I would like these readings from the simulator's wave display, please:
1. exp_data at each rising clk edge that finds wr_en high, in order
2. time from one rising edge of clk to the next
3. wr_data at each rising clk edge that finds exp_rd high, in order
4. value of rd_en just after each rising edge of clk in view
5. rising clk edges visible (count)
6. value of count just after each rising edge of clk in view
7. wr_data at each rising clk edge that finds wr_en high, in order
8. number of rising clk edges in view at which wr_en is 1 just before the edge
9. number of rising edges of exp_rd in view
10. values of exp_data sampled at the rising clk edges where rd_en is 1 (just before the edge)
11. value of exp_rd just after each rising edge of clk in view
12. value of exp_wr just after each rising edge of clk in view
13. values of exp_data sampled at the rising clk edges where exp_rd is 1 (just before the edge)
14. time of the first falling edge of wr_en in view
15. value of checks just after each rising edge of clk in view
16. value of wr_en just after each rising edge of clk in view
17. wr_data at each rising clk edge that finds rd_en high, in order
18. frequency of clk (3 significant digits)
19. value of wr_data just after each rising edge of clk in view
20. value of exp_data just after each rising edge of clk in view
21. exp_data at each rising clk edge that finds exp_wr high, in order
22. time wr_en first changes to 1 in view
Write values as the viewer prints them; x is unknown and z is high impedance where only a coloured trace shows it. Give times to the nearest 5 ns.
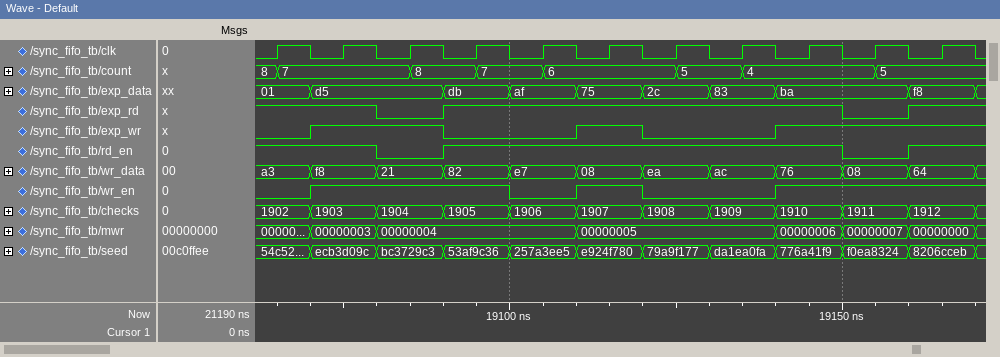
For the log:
d5, d5, db, 75, ba, ba, f8
10 ns
a3, f8, 82, e7, 08, ea, ac, 76, 64
1 1 0 1 1 1 1 1 1 0 1
11
7, 7, 8, 7, 6, 6, 5, 4, 4, 5, 5
f8, 21, 82, 08, 76, 08, 64
7
2
01, d5, db, af, 75, 2c, 83, ba, f8
1 1 0 1 1 1 1 1 1 0 1
0 1 1 0 0 1 0 0 1 1 1
01, d5, db, af, 75, 2c, 83, ba, f8
19100 ns
1902, 1903, 1904, 1905, 1906, 1907, 1908, 1909, 1910, 1911, 1912
0 1 1 1 0 1 0 0 1 1 1
a3, f8, 82, e7, 08, ea, ac, 76, 64
100 MHz
a3, f8, 21, 82, e7, 08, ea, ac, 76, 08, 64
01, d5, d5, db, af, 75, 2c, 83, ba, ba, f8
d5, d5, 75, ba, ba, f8
19070 ns
